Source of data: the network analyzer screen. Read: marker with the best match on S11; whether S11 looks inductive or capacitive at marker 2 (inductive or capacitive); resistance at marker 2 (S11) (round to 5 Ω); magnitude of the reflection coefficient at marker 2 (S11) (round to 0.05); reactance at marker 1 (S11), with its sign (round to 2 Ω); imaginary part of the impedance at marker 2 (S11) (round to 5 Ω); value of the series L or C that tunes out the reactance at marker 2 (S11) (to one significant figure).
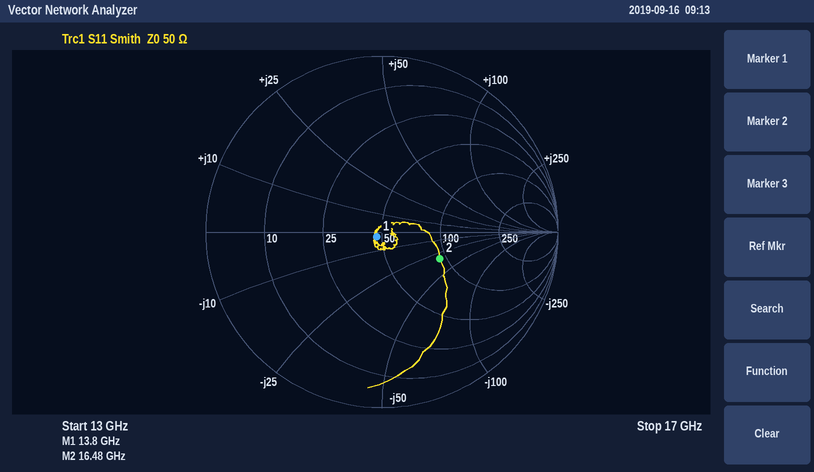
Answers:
marker 1
capacitive
90 Ω
0.35
-2 Ω
-30 Ω
300 pH
